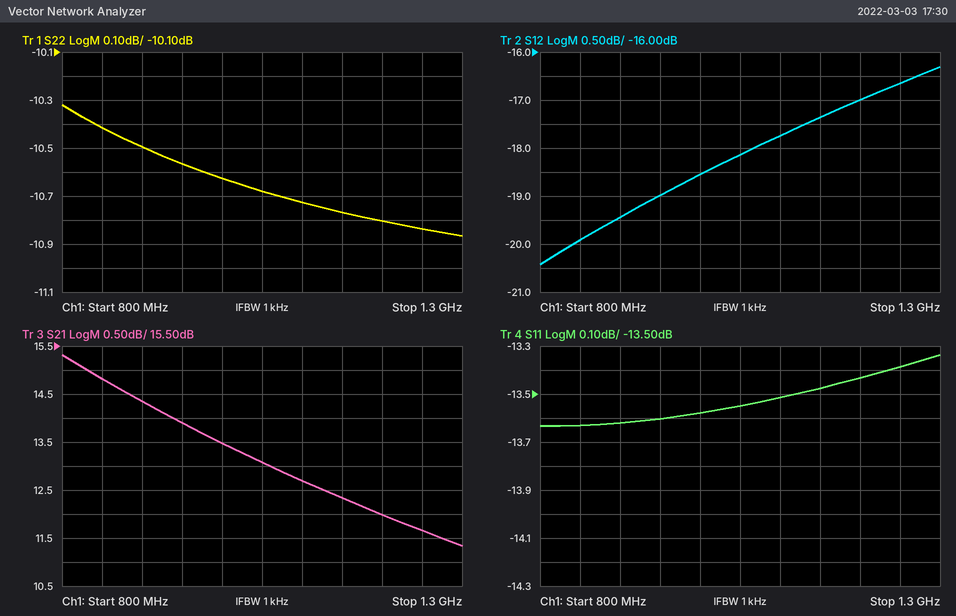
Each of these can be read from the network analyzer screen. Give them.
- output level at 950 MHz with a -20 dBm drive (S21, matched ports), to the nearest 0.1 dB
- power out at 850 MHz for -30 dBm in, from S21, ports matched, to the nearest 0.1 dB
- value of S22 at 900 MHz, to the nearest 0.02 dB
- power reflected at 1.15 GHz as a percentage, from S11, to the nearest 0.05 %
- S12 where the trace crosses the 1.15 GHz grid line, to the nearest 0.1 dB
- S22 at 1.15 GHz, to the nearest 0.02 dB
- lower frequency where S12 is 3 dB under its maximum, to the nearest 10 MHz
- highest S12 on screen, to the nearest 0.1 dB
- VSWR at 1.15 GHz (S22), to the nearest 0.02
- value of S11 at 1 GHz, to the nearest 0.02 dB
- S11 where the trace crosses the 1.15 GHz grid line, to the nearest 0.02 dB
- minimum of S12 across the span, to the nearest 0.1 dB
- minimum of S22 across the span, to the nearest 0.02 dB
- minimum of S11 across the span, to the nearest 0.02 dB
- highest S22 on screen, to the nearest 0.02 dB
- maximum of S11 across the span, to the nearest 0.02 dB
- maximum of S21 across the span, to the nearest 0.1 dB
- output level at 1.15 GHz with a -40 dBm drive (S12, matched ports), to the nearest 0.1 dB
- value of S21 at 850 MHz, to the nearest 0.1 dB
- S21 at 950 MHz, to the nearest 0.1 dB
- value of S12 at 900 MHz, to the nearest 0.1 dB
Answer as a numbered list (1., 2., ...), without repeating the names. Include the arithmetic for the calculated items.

1. -20 dBm + (13.9 dB) = -6.1 dBm
2. -30 dBm + (14.8 dB) = -15.2 dBm
3. -10.50 dB
4. 10^(-13.48/10) ≈ 4.49 %, so 4.50 % to the nearest 0.05 %
5. -17.4 dB
6. -10.76 dB
7. 910 MHz
8. -16.3 dB
9. |Γ| = 10^(-10.76/20) = 0.2897; VSWR = (1 + 0.2897)/(1 − 0.2897) ≈ 1.82
10. -13.58 dB
11. -13.48 dB
12. -20.4 dB
13. -10.86 dB
14. -13.64 dB
15. -10.32 dB
16. -13.34 dB
17. 15.3 dB
18. -40 dBm + (-17.4 dB) = -57.4 dBm
19. 14.8 dB
20. 13.9 dB
21. -19.4 dB
